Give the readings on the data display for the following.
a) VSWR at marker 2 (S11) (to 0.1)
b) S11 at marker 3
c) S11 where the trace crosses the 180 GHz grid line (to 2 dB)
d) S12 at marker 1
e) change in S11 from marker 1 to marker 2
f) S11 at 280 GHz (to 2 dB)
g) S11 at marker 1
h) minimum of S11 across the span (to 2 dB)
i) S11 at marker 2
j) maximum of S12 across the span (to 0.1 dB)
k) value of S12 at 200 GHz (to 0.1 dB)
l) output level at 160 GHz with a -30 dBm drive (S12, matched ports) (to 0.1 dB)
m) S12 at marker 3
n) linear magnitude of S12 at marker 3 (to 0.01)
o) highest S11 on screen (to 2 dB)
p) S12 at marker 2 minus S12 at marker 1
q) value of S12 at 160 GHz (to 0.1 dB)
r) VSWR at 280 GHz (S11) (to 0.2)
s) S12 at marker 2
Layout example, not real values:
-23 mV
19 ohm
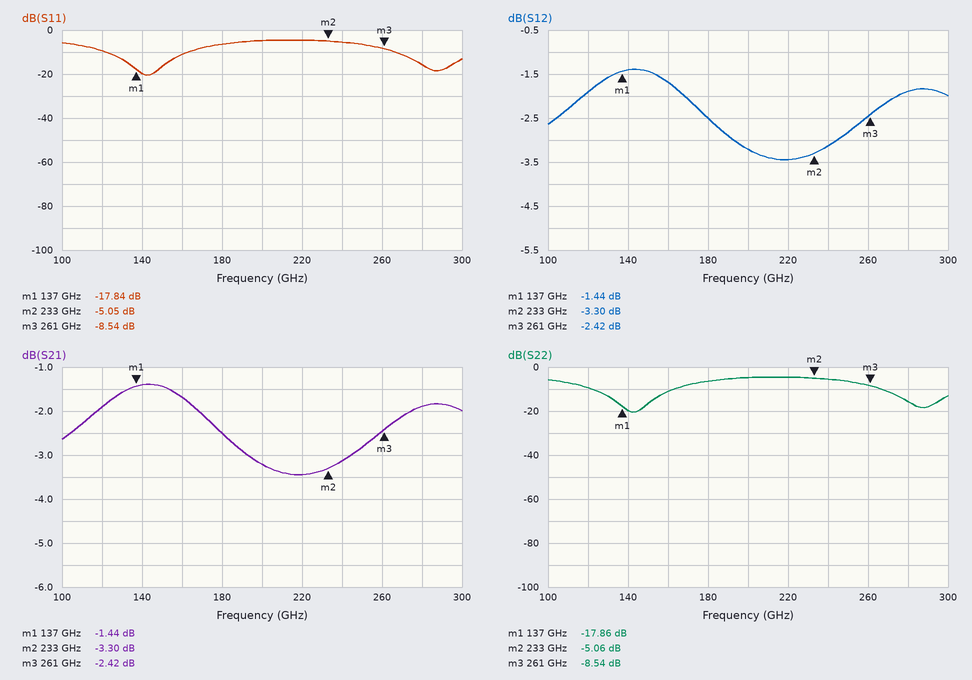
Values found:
3.5
-8.54 dB
-6 dB
-1.44 dB
12.79 dB
-16 dB
-17.84 dB
-20 dB
-5.05 dB
-1.4 dB
-3.2 dB
-31.7 dBm
-2.42 dB
0.76
-4 dB
-1.86 dB
-1.7 dB
1.4
-3.30 dB
